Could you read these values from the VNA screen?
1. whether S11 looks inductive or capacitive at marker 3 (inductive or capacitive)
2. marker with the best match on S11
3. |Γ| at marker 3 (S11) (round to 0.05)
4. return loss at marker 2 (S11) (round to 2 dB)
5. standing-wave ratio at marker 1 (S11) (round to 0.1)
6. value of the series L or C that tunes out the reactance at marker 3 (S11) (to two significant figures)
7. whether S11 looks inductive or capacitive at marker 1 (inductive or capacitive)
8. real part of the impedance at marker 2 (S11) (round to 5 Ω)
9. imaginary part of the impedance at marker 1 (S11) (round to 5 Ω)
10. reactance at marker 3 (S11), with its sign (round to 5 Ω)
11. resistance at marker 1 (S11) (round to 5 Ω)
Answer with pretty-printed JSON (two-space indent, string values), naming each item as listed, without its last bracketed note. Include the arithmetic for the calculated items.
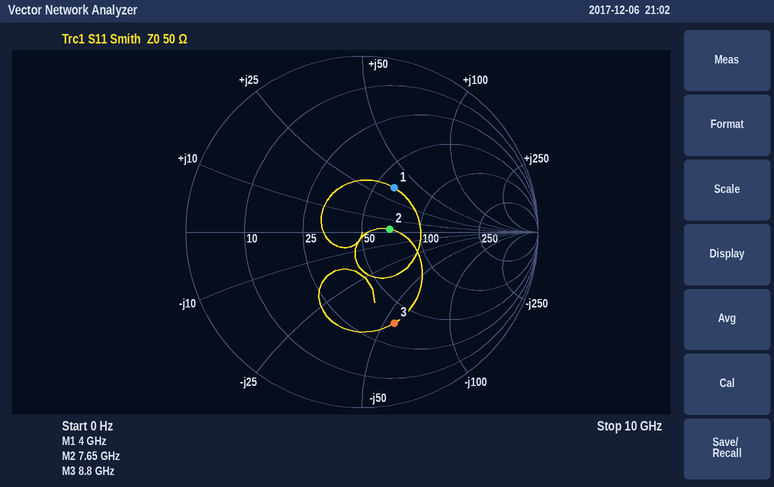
{
  "whether S11 looks inductive or capacitive at marker 3": "capacitive",
  "marker with the best match on S11": "marker 2",
  "|Γ| at marker 3 (S11)": "0.55",
  "return loss at marker 2 (S11)": "16 dB",
  "standing-wave ratio at marker 1 (S11)": "1.9",
  "value of the series L or C that tunes out the reactance at marker 3 (S11)": "L = 55 Ω/(2π × 8.8 GHz) ≈ 1.0 nH",
  "whether S11 looks inductive or capacitive at marker 1": "inductive",
  "real part of the impedance at marker 2 (S11)": "70 Ω",
  "imaginary part of the impedance at marker 1 (S11)": "+35 Ω",
  "reactance at marker 3 (S11), with its sign": "-55 Ω",
  "resistance at marker 1 (S11)": "60 Ω"
}
